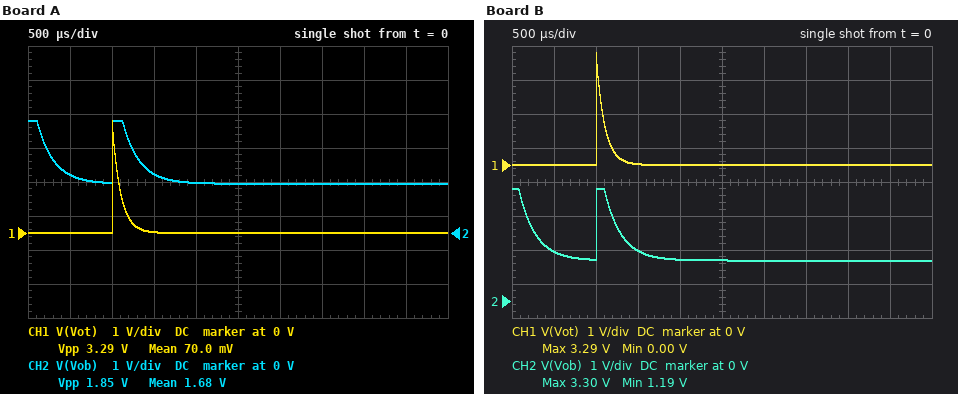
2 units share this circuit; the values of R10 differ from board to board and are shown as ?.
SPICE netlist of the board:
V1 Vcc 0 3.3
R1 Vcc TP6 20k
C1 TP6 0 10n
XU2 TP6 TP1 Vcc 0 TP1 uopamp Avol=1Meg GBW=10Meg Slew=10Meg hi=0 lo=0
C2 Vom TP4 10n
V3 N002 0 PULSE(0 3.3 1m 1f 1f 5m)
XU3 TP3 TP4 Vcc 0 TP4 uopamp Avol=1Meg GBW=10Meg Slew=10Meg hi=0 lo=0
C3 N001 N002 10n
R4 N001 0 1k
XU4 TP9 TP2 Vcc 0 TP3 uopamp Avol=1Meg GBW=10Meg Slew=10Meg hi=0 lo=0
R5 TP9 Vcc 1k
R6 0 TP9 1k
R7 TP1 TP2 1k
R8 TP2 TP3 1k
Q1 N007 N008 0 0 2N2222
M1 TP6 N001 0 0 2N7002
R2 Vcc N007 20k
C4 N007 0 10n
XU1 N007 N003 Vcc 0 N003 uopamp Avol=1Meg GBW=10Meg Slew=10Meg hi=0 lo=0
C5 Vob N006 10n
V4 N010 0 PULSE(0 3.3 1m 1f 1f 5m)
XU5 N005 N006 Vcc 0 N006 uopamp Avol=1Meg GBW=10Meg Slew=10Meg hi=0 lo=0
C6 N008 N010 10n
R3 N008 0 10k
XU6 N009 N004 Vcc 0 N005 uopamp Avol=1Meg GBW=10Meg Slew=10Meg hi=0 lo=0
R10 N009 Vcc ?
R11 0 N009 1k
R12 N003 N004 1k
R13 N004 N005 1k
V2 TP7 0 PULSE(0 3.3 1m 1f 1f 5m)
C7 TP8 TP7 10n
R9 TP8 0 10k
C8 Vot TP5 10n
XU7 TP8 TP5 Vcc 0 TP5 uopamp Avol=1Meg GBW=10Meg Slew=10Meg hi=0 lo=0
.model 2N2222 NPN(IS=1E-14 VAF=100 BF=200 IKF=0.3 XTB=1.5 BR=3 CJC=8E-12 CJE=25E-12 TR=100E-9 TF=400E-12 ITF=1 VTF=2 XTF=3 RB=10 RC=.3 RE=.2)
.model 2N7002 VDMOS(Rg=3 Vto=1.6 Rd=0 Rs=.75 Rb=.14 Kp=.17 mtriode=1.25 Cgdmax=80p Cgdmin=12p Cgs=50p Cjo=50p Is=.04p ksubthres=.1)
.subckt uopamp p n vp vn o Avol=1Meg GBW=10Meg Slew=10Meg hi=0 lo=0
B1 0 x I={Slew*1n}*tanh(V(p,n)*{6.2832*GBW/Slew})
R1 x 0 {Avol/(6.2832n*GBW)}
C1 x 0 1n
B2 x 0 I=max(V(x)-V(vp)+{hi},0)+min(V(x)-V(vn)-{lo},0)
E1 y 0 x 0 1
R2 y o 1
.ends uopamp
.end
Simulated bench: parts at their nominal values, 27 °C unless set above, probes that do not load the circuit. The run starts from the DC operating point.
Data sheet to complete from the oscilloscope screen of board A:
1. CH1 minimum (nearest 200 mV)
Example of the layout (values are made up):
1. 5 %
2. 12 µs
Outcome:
1. 0 V
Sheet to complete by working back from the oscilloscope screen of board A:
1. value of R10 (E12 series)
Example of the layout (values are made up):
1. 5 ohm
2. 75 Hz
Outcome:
1. 390 Ω
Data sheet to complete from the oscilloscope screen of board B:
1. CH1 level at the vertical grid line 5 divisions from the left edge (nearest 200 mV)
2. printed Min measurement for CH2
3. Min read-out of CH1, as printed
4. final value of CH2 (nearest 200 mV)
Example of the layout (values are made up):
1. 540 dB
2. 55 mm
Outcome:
1. 0 V
2. 1.19 V
3. 0.00 V
4. 1.2 V
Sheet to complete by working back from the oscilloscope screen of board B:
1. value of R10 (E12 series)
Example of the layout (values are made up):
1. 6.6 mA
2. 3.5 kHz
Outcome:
1. 470 Ω
